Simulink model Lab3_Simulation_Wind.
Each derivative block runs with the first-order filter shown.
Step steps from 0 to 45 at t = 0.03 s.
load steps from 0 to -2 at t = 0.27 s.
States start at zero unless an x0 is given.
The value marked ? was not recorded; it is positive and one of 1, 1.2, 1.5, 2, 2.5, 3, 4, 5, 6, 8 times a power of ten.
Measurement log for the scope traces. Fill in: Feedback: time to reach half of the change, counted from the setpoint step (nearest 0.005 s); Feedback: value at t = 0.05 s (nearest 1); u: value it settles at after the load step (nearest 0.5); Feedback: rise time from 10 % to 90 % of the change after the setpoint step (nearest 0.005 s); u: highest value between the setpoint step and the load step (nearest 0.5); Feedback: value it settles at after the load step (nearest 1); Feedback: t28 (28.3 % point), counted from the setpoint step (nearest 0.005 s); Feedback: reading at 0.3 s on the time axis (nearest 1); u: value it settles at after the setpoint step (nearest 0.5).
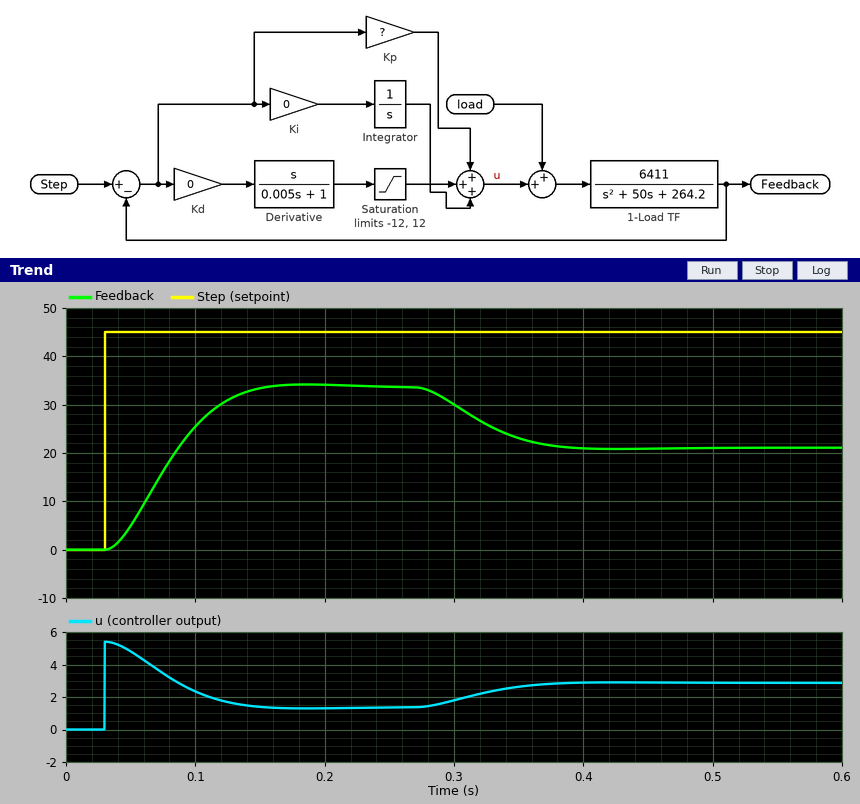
0.045 s
5
3.0
0.075 s
5.5
21
0.030 s
30
1.5
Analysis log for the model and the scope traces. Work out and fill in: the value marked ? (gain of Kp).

0.12
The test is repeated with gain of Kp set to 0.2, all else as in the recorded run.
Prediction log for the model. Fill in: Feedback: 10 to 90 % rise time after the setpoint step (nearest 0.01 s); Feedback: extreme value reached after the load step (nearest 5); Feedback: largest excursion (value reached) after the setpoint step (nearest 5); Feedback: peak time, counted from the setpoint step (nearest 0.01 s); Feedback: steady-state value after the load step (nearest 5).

0.05 s
30
40
0.10 s
30
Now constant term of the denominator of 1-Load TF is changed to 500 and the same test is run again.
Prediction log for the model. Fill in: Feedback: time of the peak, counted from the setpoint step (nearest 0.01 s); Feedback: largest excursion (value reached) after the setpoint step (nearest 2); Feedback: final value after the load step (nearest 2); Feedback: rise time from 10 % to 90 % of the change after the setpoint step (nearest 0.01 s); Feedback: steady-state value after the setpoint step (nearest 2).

0.12 s
28
18
0.06 s
28
